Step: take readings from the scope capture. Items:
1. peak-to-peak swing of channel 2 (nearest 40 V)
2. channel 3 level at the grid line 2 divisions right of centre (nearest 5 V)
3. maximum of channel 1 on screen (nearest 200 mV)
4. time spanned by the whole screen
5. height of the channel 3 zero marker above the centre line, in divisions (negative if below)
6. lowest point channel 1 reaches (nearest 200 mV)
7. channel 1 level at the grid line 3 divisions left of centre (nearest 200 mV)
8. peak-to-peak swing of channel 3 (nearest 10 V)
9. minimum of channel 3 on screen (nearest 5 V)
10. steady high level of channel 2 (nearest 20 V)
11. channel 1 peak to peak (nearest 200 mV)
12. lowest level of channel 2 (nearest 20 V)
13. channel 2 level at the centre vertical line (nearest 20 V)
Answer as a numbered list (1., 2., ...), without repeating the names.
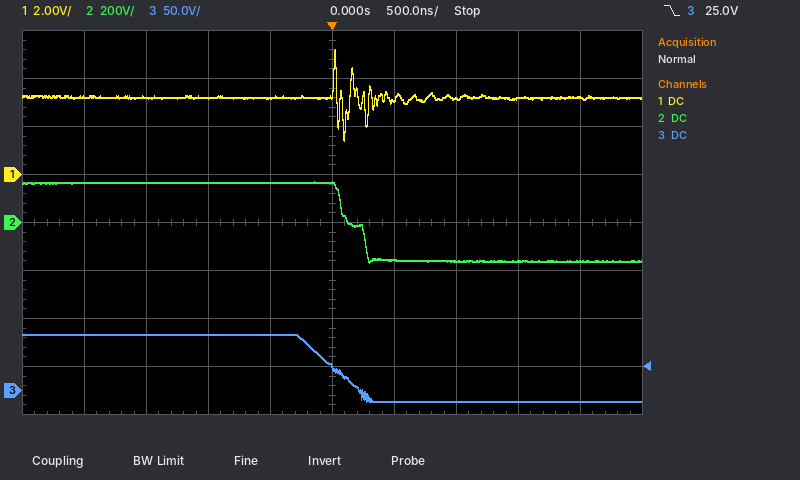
1. 320 V
2. -10 V
3. 5.2 V
4. 5 µs
5. -3.5 div
6. 1.4 V
7. 3.2 V
8. 70 V
9. -10 V
10. 160 V
11. 3.8 V
12. -160 V
13. 160 V
